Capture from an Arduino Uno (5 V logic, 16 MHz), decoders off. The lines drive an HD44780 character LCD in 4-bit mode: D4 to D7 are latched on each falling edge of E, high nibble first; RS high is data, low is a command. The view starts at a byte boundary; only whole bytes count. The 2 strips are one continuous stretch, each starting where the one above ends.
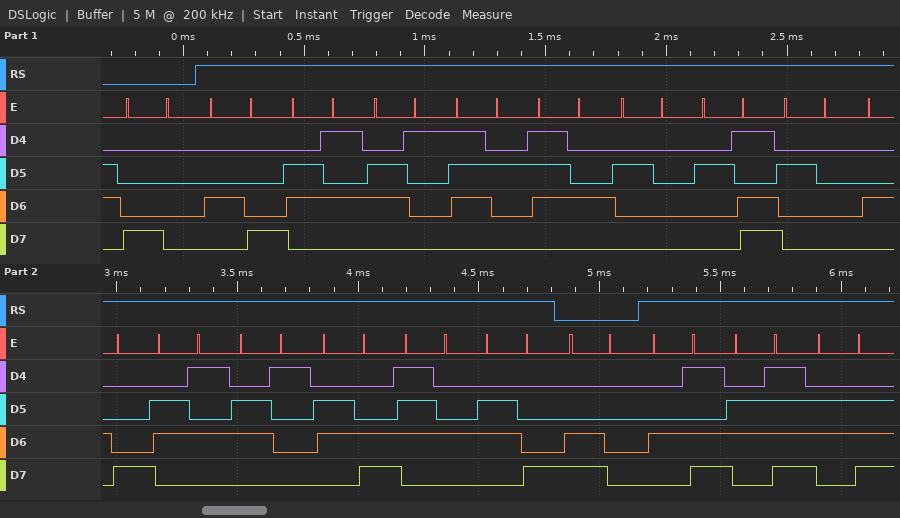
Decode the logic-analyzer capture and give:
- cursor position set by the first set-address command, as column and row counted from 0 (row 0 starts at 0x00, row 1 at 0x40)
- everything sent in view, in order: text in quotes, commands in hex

column 0, row 0
0x80 "Heart - Health" 0xC0 "Mon"
